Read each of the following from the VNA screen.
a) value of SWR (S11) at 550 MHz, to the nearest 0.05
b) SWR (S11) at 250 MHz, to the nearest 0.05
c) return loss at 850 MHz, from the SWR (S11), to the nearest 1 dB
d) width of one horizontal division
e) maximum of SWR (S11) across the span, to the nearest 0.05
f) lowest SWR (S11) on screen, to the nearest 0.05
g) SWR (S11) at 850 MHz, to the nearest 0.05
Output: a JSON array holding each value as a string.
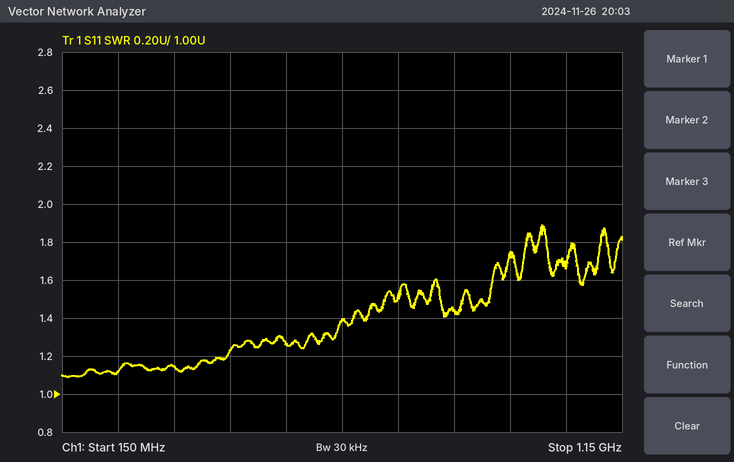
["1.25", "1.10", "15 dB", "100 MHz", "1.90", "1.10", "1.45"]
